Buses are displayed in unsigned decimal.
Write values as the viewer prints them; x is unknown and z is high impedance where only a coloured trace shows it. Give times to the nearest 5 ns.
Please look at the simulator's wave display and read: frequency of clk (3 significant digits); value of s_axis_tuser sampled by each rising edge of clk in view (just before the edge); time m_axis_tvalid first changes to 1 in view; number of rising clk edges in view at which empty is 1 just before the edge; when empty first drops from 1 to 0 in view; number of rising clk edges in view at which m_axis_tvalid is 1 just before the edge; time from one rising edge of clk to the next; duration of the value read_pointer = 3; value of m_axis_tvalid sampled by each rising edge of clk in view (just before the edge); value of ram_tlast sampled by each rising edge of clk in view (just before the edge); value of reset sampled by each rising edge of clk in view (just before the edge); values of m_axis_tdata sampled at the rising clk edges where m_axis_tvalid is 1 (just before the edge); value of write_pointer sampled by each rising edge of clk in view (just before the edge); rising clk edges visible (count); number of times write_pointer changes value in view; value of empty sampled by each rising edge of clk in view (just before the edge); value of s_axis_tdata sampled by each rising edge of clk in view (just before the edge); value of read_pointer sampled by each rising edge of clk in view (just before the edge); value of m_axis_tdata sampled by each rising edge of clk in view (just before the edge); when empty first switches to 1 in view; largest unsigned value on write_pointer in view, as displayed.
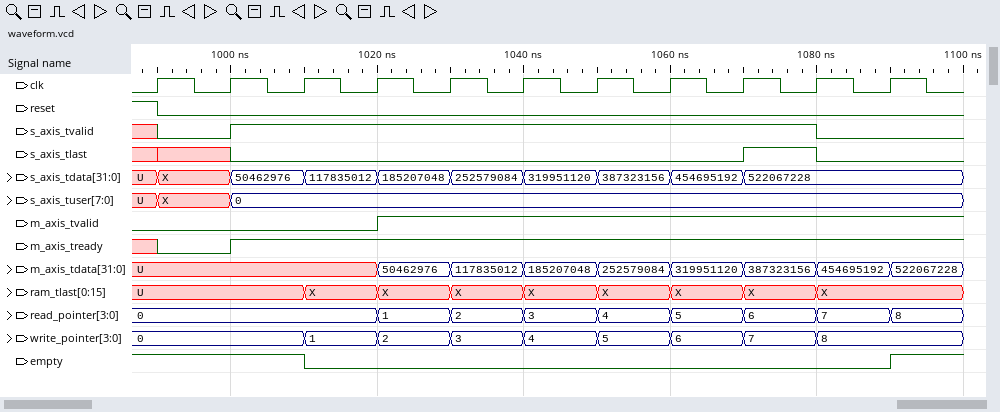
100 MHz
U, X, 0, 0, 0, 0, 0, 0, 0, 0, 0
1020 ns
3
1010 ns
7
10 ns
10 ns
0 0 0 0 1 1 1 1 1 1 1
U, U, U, X, X, X, X, X, X, X, X
1 0 0 0 0 0 0 0 0 0 0
50462976, 117835012, 185207048, 252579084, 319951120, 387323156, 454695192
0, 0, 0, 1, 2, 3, 4, 5, 6, 7, 8
11
8
1 1 1 0 0 0 0 0 0 0 0
U, X, 50462976, 117835012, 185207048, 252579084, 319951120, 387323156, 454695192, 522067228, 522067228
0, 0, 0, 0, 1, 2, 3, 4, 5, 6, 7
U, U, U, U, 50462976, 117835012, 185207048, 252579084, 319951120, 387323156, 454695192
1090 ns
8
